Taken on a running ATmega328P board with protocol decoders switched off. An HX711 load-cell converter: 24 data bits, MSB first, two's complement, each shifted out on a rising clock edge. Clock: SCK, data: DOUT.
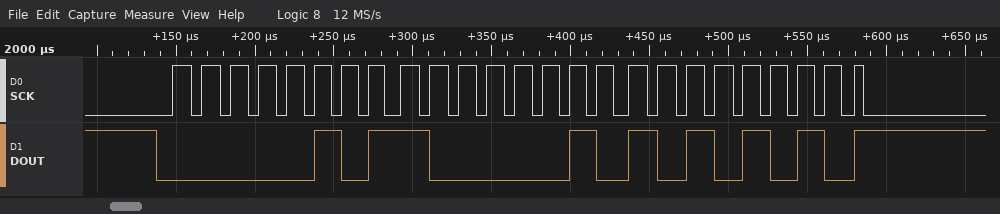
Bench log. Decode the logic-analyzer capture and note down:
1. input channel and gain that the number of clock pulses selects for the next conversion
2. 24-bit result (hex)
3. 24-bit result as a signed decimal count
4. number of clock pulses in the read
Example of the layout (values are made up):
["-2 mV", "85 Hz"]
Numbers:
["channel A, gain 128", "0x0582AA", "361130", "25"]
